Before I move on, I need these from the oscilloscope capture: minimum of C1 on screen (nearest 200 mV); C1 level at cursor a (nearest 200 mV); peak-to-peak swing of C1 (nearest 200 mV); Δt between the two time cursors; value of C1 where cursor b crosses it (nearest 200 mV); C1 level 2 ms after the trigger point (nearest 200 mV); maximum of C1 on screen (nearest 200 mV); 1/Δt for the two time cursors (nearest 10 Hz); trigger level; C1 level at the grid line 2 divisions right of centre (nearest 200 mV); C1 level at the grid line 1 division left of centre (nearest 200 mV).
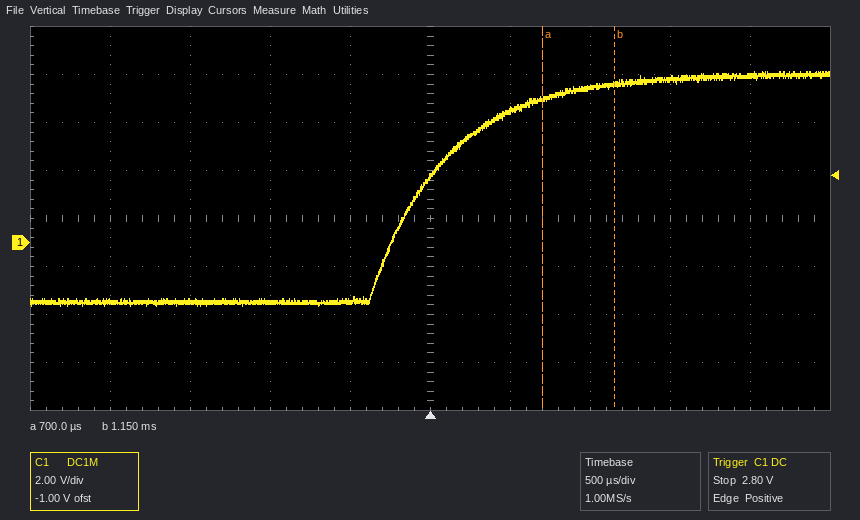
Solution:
-2.6 V
6.0 V
9.8 V
450 µs
6.6 V
7.0 V
7.2 V
2.22 kHz
2.80 V
6.4 V
-2.4 V
